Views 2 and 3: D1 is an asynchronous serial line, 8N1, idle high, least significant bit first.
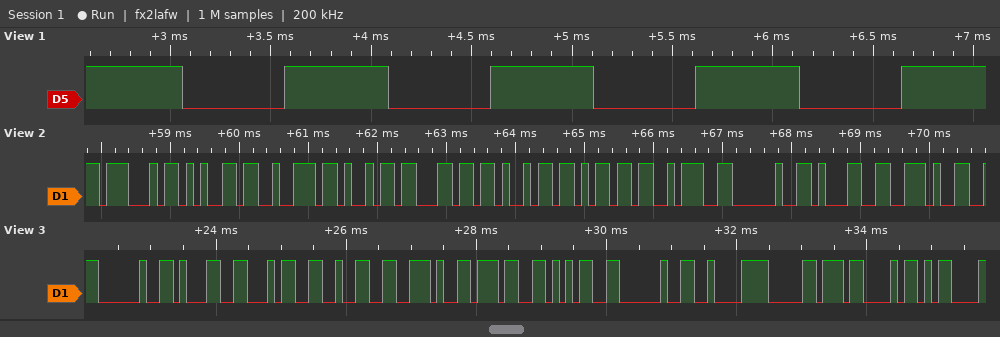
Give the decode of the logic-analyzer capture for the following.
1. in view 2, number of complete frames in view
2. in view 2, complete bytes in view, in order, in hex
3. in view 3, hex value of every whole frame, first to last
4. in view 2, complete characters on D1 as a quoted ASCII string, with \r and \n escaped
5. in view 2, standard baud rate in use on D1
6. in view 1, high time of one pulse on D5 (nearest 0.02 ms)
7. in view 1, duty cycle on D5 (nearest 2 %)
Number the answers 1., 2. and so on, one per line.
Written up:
1. 11
2. 47 65 72 69 6C 69 6D 3A 20 31 2E
3. 20 31 34 32 2E 37 35 20 C2 B0 43 0D
4. "Gerilim: 1."
5. 9600 baud
6. 0.52 ms
7. 50 %
